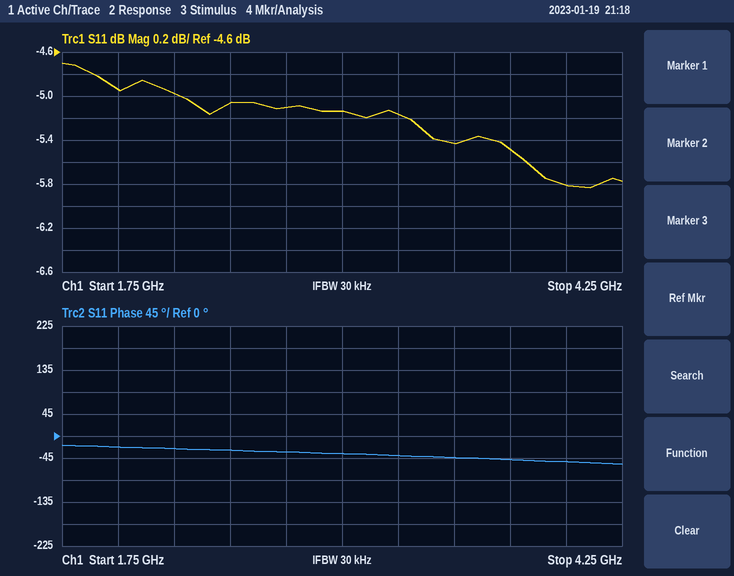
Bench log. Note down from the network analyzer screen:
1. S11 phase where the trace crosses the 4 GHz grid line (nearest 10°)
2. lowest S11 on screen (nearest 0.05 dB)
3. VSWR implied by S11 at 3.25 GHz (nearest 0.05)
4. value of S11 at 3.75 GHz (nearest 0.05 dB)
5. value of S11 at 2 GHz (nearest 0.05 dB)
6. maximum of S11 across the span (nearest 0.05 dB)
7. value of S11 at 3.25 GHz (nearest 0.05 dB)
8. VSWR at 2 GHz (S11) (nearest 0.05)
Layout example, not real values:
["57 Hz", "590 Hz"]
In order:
["-50°", "-5.85 dB", "3.45", "-5.50 dB", "-4.95 dB", "-4.70 dB", "-5.15 dB", "3.60"]
